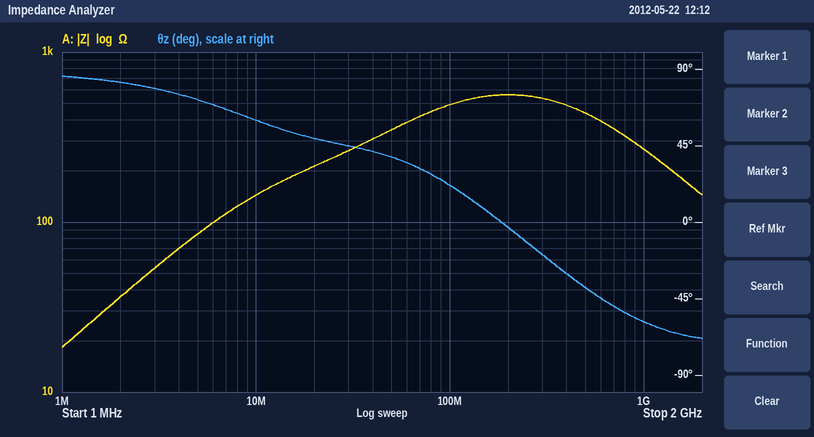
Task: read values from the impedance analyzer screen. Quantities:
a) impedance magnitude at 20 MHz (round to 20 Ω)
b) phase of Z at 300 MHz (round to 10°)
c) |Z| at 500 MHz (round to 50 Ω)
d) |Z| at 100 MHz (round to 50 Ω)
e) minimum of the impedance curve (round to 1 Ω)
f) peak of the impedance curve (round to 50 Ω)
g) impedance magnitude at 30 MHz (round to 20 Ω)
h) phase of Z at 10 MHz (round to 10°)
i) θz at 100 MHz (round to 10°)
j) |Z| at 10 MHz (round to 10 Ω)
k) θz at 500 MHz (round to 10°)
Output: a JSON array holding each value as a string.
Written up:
["220 Ω", "-20°", "450 Ω", "500 Ω", "18 Ω", "550 Ω", "260 Ω", "60°", "20°", "140 Ω", "-40°"]
